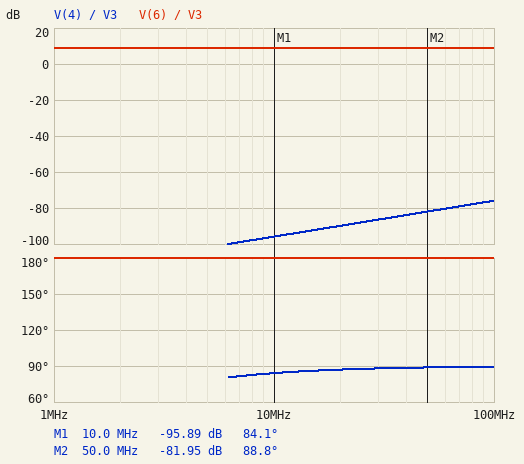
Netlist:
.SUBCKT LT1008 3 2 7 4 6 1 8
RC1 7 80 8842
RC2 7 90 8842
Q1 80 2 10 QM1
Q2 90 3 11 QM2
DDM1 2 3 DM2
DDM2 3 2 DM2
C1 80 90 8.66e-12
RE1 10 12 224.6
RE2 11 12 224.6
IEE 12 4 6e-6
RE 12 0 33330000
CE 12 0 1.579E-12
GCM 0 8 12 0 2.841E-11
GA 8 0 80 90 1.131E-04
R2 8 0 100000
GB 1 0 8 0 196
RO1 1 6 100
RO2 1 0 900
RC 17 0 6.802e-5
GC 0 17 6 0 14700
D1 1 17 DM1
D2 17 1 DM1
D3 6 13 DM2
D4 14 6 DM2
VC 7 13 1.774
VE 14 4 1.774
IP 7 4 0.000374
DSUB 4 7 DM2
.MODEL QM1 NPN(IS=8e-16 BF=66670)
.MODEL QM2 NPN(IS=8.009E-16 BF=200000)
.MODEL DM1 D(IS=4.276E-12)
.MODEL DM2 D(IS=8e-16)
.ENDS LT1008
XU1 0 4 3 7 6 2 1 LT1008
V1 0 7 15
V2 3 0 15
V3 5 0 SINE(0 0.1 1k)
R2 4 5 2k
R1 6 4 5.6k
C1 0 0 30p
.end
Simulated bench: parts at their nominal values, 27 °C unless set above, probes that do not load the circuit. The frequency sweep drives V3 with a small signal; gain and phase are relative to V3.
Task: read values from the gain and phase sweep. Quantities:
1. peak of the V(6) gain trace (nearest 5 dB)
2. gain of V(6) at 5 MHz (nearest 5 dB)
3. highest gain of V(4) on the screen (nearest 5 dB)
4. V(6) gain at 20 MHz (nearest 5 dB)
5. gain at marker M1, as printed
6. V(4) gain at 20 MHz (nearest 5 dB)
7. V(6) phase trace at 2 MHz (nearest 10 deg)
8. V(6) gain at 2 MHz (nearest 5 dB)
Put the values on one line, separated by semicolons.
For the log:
10 dB; 10 dB; -75 dB; 10 dB; -95.89 dB; -90 dB; 180 deg; 10 dB
